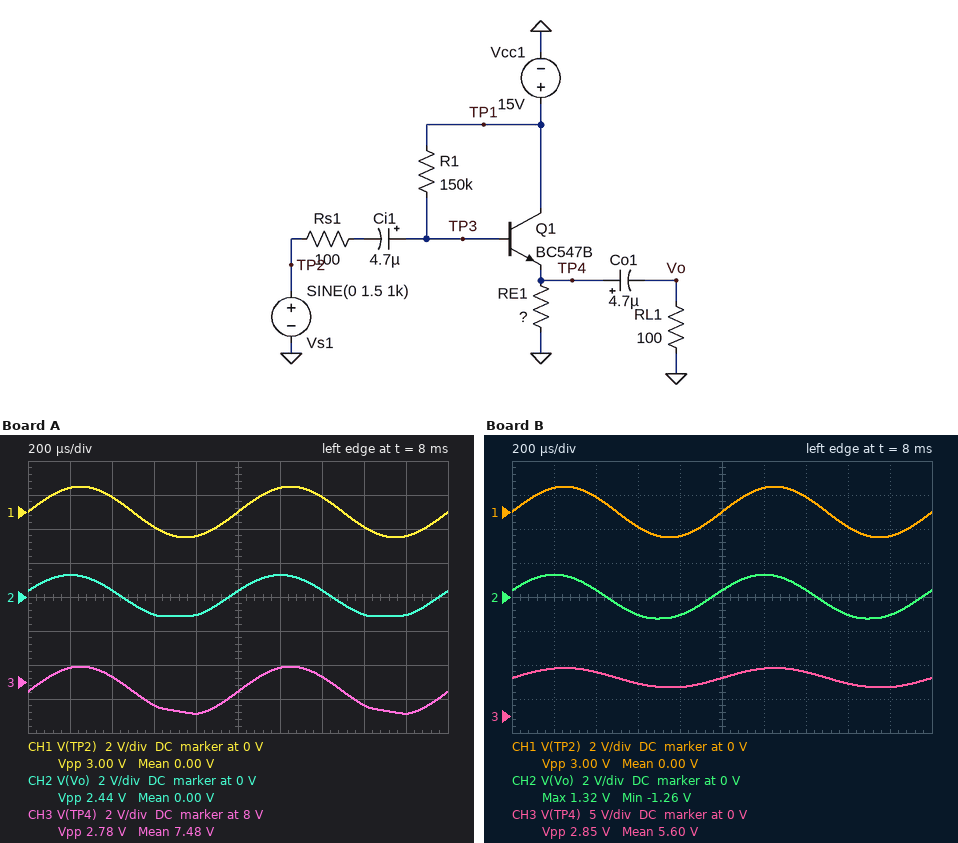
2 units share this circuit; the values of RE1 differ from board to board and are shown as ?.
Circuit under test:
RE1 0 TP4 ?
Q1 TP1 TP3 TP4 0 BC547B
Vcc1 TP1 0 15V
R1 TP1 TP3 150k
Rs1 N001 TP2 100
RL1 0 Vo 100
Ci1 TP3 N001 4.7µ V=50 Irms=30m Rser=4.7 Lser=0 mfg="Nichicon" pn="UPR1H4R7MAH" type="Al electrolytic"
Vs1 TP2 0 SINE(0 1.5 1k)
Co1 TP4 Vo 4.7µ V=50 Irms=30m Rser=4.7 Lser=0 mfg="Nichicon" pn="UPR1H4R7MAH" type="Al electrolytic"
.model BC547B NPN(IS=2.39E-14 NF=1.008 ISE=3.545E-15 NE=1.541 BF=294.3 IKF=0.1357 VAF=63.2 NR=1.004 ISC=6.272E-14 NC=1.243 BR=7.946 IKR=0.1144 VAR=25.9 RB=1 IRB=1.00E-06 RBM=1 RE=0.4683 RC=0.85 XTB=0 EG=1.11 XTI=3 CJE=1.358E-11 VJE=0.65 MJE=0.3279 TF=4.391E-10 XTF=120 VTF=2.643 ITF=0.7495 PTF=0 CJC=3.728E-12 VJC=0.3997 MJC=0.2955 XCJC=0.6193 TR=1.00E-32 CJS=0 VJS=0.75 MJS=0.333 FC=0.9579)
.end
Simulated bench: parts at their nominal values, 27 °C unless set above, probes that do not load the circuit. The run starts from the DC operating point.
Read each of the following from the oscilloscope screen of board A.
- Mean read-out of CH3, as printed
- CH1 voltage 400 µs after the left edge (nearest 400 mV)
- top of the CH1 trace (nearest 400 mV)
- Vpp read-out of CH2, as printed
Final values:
7.48 V
800 mV
1.6 V
2.44 V
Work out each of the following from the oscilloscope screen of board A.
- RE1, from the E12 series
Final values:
560 Ω
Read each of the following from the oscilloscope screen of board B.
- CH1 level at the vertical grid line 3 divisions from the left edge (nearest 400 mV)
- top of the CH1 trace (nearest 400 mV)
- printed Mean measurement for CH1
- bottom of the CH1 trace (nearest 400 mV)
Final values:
-800 mV
1.6 V
0.00 V
-1.6 V
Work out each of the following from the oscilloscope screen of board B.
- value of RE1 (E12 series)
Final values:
330 Ω
